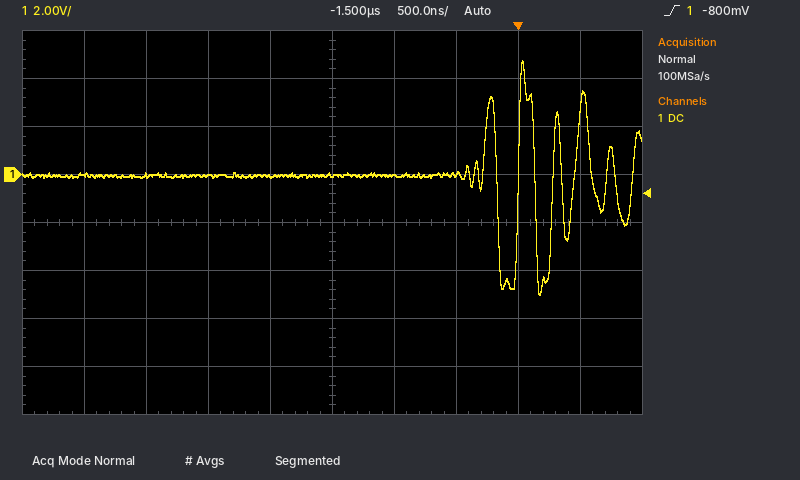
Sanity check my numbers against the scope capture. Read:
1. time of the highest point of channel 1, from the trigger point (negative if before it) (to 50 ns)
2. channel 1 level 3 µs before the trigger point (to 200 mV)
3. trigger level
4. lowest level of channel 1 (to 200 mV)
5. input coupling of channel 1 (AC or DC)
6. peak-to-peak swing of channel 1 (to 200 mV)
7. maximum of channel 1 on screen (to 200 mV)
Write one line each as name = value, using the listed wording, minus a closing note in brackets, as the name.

time of the highest point of channel 1, from the trigger point (negative if before it) = +50 ns
channel 1 level 3 µs before the trigger point = 0.0 V
trigger level = -800 mV
lowest level of channel 1 = -5.0 V
input coupling of channel 1 = DC
peak-to-peak swing of channel 1 = 9.8 V
maximum of channel 1 on screen = 4.8 V
